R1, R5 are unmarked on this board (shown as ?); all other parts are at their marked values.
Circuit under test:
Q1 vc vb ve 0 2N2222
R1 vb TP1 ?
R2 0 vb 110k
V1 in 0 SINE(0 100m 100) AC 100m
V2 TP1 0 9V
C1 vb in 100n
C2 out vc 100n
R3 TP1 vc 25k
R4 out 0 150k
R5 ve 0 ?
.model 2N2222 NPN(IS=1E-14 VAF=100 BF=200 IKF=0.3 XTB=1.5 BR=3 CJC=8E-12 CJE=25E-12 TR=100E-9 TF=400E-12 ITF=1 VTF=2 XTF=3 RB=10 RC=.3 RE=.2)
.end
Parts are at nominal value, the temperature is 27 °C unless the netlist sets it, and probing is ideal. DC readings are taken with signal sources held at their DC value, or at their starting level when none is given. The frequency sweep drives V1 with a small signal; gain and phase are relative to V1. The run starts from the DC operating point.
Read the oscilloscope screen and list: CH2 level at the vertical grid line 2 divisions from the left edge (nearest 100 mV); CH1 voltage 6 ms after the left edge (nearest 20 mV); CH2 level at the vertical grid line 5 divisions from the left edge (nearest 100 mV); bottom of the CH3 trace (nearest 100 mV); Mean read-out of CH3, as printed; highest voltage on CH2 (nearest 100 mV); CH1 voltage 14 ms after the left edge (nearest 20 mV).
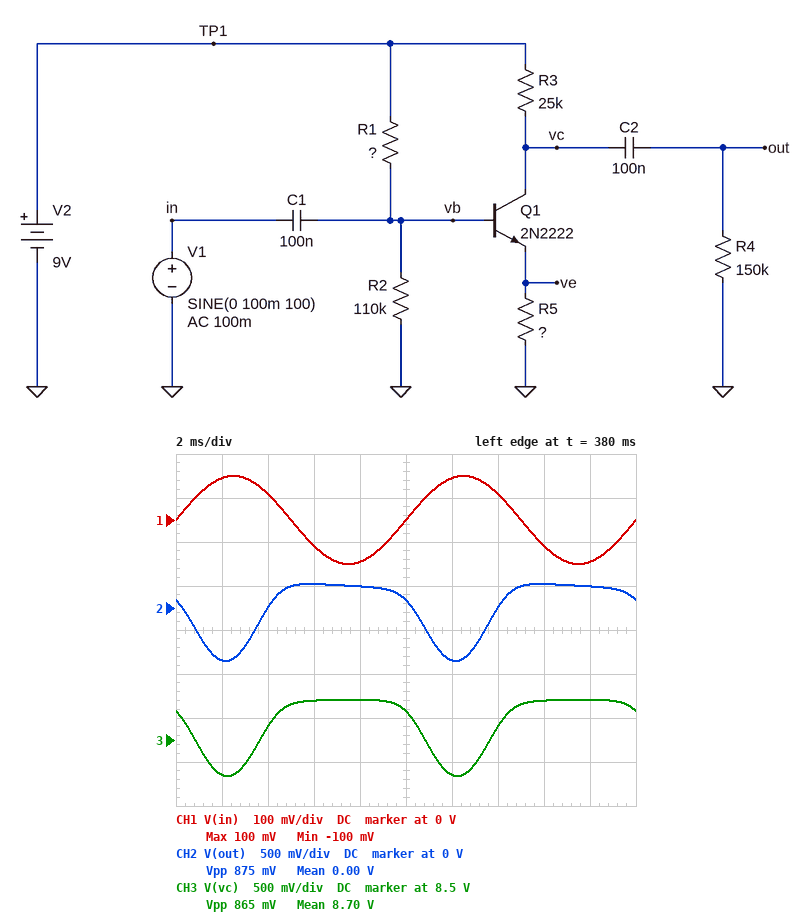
0 V
-60 mV
100 mV
8.1 V
8.70 V
300 mV
60 mV
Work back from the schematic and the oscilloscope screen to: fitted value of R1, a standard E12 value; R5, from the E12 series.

1.8 MΩ
1 kΩ
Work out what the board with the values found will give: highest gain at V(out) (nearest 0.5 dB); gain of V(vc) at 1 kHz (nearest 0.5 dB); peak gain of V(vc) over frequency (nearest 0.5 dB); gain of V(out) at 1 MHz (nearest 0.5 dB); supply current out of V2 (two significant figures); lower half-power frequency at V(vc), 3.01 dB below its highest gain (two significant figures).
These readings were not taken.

9.5 dB
9.5 dB
9.5 dB
9.0 dB
9.0 µA
15 Hz
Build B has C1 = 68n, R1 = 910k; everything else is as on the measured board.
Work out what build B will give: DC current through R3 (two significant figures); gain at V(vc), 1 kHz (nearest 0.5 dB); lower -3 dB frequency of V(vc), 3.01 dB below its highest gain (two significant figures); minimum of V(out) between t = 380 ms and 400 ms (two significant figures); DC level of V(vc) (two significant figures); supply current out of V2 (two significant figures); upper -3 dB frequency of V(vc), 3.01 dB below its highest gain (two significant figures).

240 µA
25.5 dB
34 Hz
-1.8 V
3.1 V
250 µA
1.5 MHz
